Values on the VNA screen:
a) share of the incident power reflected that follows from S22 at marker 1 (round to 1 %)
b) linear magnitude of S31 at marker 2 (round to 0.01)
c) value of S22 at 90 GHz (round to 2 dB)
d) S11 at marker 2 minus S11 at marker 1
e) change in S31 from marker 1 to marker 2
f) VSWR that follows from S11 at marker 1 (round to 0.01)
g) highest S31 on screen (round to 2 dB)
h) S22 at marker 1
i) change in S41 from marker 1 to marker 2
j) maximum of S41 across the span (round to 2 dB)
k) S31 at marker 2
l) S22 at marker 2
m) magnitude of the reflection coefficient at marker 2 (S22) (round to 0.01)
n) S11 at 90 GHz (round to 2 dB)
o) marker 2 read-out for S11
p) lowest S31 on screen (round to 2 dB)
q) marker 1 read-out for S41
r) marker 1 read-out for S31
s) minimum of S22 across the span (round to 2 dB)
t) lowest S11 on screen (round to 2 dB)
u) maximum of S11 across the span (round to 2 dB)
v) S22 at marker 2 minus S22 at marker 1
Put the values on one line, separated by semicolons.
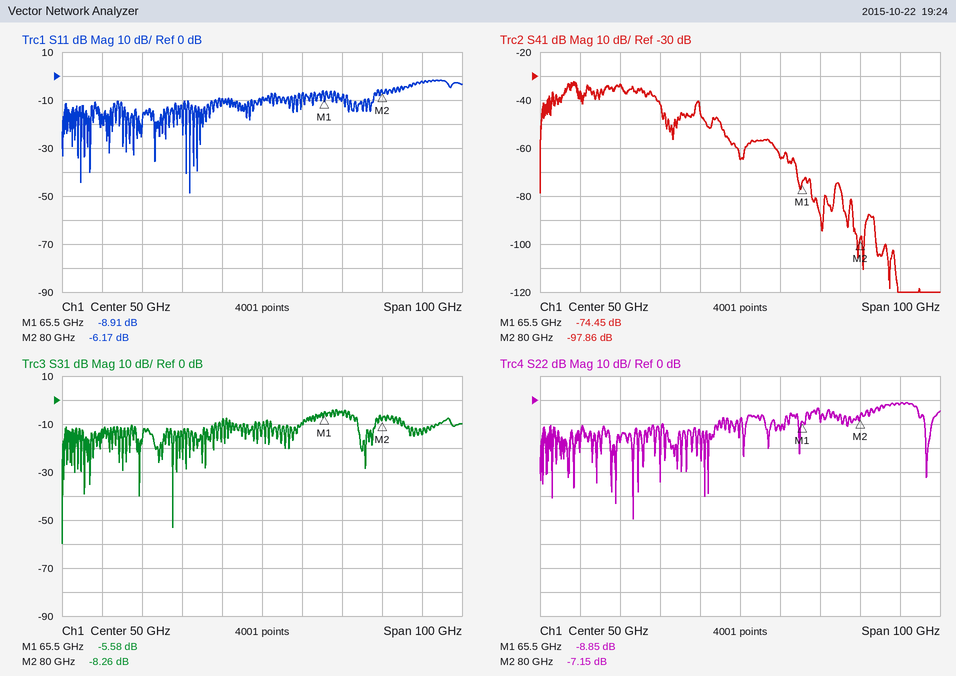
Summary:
13 %; 0.39; -2 dB; 2.74 dB; -2.68 dB; 2.12; -4 dB; -8.85 dB; -23.41 dB; -32 dB; -8.26 dB; -7.15 dB; 0.44; -2 dB; -6.17 dB; -60 dB; -74.45 dB; -5.58 dB; -50 dB; -48 dB; -2 dB; 1.70 dB
